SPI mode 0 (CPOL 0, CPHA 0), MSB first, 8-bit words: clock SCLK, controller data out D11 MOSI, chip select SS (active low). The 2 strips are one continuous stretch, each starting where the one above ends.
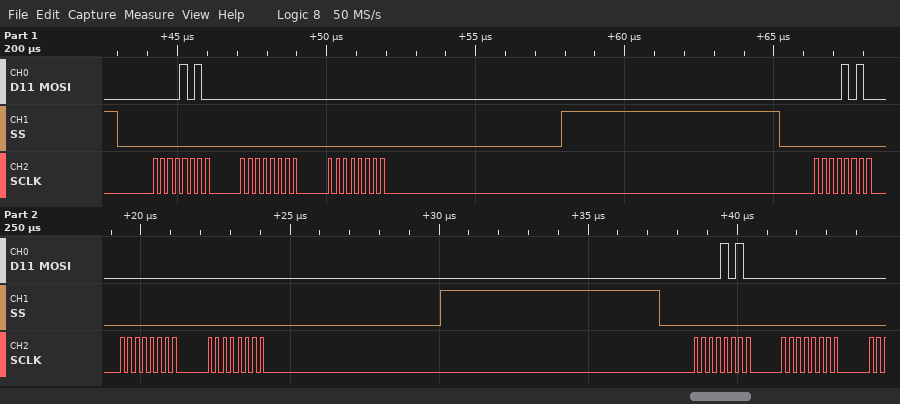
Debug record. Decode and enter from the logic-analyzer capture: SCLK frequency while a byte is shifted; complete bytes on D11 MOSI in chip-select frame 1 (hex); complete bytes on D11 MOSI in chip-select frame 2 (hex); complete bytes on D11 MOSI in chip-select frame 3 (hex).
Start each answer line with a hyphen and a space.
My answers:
- 4 MHz
- 0A 00 00
- 0A 00 00
- 0A 00
